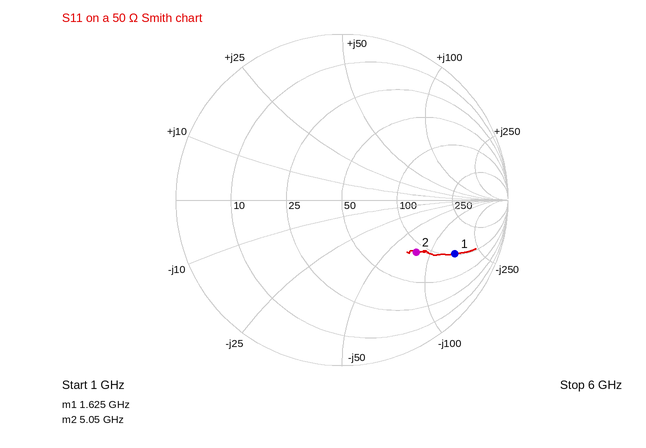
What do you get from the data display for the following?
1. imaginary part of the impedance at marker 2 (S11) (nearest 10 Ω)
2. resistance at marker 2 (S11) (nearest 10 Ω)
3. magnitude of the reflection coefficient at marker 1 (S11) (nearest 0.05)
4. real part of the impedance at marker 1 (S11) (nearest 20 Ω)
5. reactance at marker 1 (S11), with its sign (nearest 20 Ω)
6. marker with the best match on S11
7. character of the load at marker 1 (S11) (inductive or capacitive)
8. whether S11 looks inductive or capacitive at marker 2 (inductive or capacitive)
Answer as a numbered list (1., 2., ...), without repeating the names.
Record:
1. -80 Ω
2. 90 Ω
3. 0.75
4. 100 Ω
5. -160 Ω
6. marker 2
7. capacitive
8. capacitive
